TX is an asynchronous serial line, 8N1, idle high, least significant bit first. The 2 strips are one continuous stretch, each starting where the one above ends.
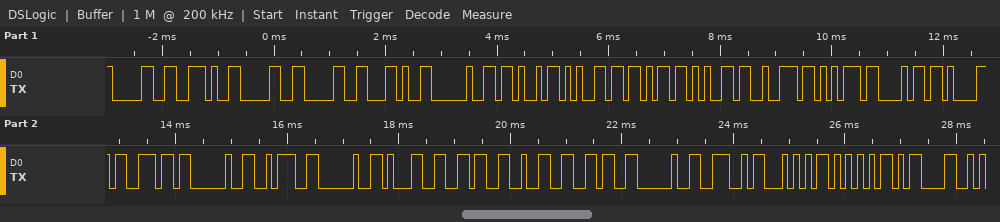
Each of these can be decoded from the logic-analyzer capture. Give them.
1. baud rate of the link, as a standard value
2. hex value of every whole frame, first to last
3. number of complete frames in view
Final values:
9600 baud
30 2E 30 30 2C 20 4B 65 6B 65 72 75 68 61 6E 20 3A 20 31 36 32 36 20 4E 54 55 0D
27
